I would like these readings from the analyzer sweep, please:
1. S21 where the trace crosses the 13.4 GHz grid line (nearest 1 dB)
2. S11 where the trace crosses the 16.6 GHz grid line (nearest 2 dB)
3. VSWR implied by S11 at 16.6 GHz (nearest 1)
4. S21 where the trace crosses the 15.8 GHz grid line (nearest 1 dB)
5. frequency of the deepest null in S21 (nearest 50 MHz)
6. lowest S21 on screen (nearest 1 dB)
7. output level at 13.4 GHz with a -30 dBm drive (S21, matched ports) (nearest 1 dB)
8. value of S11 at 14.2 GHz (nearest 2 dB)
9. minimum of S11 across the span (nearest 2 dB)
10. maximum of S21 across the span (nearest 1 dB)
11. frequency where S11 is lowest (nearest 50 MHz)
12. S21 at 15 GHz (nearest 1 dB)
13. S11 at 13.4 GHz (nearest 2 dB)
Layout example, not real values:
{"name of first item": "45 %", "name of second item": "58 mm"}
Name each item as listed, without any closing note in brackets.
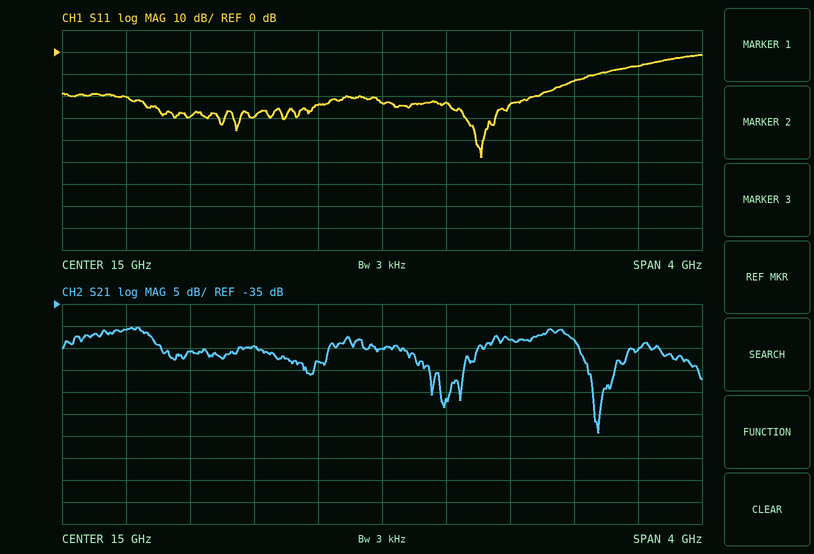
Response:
{"S21 where the trace crosses the 13.4 GHz grid line": "-41 dB", "S11 where the trace crosses the 16.6 GHz grid line": "-6 dB", "VSWR implied by S11 at 16.6 GHz": "3", "S21 where the trace crosses the 15.8 GHz grid line": "-43 dB", "frequency of the deepest null in S21": "16.35 GHz", "lowest S21 on screen": "-64 dB", "output level at 13.4 GHz with a -30 dBm drive (S21, matched ports)": "-71 dBm", "value of S11 at 14.2 GHz": "-30 dB", "minimum of S11 across the span": "-48 dB", "maximum of S21 across the span": "-40 dB", "frequency where S11 is lowest": "15.60 GHz", "S21 at 15 GHz": "-45 dB", "S11 at 13.4 GHz": "-20 dB"}
